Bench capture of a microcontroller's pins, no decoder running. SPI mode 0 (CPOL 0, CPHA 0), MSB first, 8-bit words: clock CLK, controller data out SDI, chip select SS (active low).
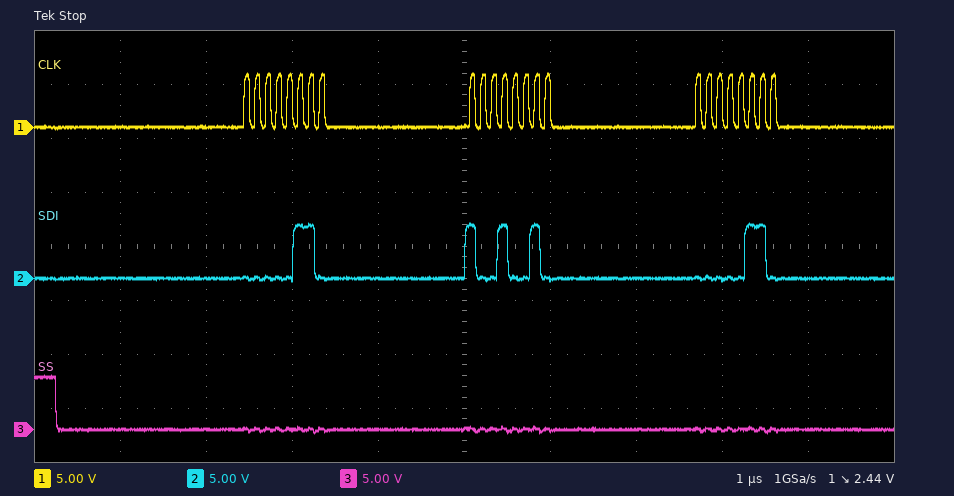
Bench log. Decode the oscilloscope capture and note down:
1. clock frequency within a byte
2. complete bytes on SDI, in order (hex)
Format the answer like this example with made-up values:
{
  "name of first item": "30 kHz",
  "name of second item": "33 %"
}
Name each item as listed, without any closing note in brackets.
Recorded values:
{
  "clock frequency within a byte": "8 MHz",
  "complete bytes on SDI, in order": "0x06 0x92 0x06"
}
